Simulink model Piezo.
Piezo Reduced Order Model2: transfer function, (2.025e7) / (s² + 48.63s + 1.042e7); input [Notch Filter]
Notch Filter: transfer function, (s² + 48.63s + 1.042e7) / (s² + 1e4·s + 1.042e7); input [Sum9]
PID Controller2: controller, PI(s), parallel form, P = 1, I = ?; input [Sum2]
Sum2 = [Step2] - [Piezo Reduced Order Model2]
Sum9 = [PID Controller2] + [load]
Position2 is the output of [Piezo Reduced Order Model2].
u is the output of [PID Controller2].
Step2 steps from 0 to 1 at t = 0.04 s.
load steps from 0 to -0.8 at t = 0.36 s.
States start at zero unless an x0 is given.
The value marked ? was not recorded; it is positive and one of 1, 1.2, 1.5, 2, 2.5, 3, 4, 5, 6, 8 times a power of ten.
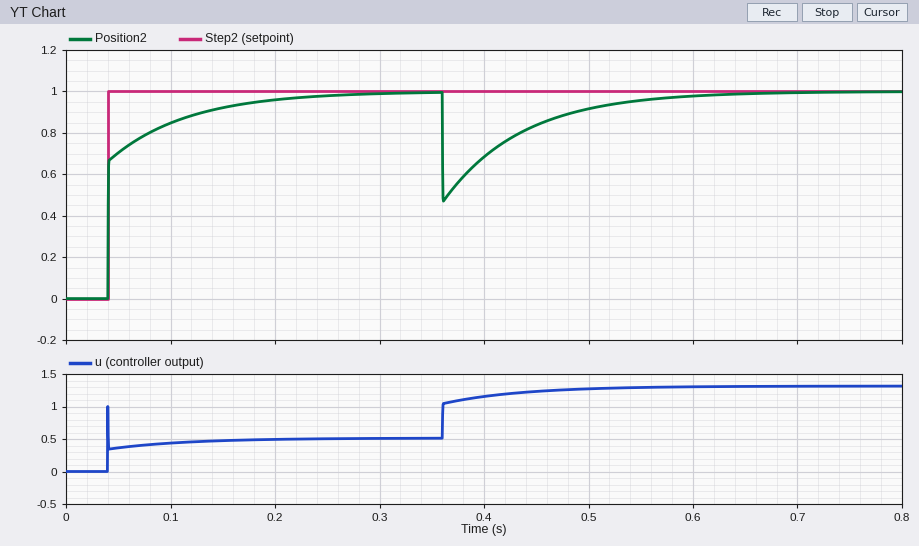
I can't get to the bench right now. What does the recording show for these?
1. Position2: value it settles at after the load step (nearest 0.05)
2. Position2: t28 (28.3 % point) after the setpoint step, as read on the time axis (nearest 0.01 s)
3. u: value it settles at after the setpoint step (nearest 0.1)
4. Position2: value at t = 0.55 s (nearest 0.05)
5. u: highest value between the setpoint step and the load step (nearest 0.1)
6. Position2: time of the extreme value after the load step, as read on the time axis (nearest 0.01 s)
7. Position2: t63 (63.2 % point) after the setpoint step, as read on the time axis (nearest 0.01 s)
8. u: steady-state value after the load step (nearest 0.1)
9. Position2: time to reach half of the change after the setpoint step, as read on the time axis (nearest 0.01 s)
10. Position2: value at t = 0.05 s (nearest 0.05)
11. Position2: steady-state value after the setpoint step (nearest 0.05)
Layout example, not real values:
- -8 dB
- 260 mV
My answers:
- 1.00
- 0.04 s
- 0.5
- 0.95
- 1.0
- 0.36 s
- 0.04 s
- 1.3
- 0.04 s
- 0.70
- 1.00
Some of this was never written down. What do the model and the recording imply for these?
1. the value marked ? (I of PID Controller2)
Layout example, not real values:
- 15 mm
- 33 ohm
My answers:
- 20
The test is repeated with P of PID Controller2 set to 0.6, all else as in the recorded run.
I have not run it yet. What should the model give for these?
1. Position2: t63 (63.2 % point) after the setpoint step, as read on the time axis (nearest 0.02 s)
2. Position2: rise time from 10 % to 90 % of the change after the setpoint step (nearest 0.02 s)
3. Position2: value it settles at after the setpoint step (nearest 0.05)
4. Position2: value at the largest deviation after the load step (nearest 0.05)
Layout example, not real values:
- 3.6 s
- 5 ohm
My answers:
- 0.06 s
- 0.08 s
- 1.00
- 0.30
